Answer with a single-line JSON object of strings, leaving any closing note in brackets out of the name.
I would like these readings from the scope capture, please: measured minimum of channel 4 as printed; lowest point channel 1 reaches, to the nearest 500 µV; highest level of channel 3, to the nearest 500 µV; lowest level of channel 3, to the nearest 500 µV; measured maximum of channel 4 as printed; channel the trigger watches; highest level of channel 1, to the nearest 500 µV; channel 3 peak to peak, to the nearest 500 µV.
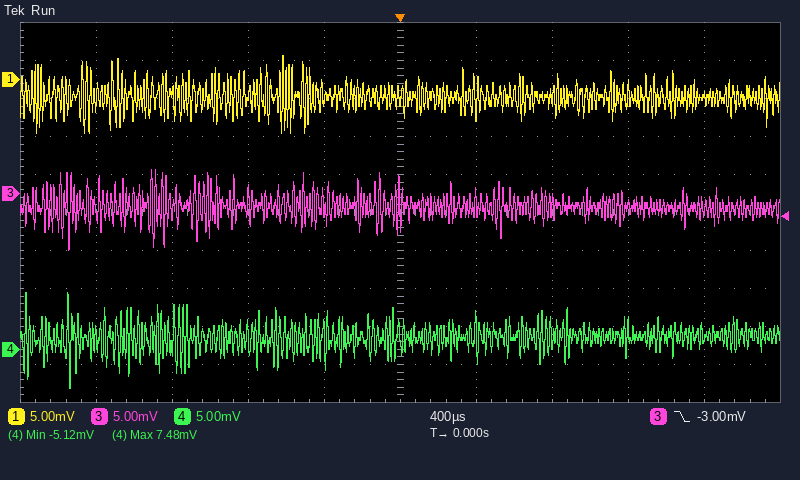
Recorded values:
{"measured minimum of channel 4 as printed": "-5.12 mV", "lowest point channel 1 reaches, to the nearest 500 µV": "-7.0 mV", "highest level of channel 3, to the nearest 500 µV": "3.0 mV", "lowest level of channel 3, to the nearest 500 µV": "-7.5 mV", "measured maximum of channel 4 as printed": "7.48 mV", "channel the trigger watches": "channel 3", "highest level of channel 1, to the nearest 500 µV": "3.0 mV", "channel 3 peak to peak, to the nearest 500 µV": "10.5 mV"}
